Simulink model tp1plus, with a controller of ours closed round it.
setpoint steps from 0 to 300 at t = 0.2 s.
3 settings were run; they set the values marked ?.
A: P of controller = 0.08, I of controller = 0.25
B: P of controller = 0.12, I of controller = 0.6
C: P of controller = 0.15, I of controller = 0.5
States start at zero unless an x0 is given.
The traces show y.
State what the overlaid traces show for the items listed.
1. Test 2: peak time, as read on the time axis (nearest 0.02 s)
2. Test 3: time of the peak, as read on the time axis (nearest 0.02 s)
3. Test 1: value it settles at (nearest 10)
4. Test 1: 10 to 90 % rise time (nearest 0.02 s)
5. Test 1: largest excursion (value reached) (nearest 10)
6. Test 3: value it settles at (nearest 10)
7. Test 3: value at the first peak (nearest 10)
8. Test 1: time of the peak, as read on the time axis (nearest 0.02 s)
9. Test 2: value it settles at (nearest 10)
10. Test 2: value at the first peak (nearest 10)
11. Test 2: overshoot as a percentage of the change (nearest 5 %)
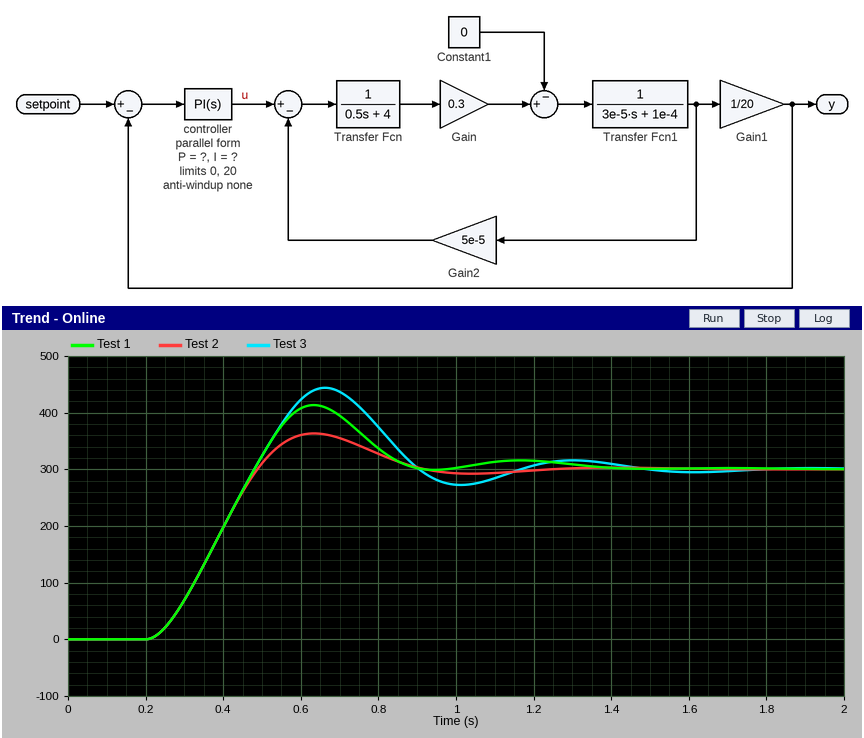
0.64 s
0.66 s
300
0.20 s
410
300
440
0.64 s
300
360
20 %
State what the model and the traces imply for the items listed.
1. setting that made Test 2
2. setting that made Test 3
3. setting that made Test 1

A
B
C
